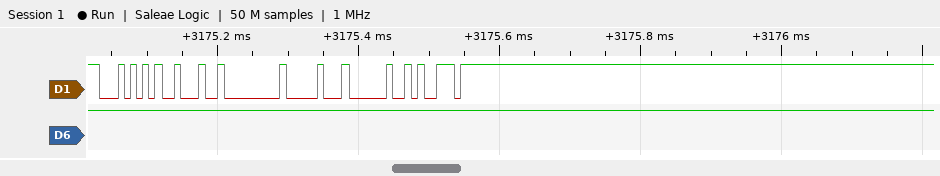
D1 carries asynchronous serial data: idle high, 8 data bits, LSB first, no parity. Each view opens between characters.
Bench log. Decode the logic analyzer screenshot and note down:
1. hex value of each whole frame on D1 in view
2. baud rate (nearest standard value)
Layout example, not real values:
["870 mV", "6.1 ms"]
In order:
["54, 22, 00, 10, 20, B9", "115200 baud"]
